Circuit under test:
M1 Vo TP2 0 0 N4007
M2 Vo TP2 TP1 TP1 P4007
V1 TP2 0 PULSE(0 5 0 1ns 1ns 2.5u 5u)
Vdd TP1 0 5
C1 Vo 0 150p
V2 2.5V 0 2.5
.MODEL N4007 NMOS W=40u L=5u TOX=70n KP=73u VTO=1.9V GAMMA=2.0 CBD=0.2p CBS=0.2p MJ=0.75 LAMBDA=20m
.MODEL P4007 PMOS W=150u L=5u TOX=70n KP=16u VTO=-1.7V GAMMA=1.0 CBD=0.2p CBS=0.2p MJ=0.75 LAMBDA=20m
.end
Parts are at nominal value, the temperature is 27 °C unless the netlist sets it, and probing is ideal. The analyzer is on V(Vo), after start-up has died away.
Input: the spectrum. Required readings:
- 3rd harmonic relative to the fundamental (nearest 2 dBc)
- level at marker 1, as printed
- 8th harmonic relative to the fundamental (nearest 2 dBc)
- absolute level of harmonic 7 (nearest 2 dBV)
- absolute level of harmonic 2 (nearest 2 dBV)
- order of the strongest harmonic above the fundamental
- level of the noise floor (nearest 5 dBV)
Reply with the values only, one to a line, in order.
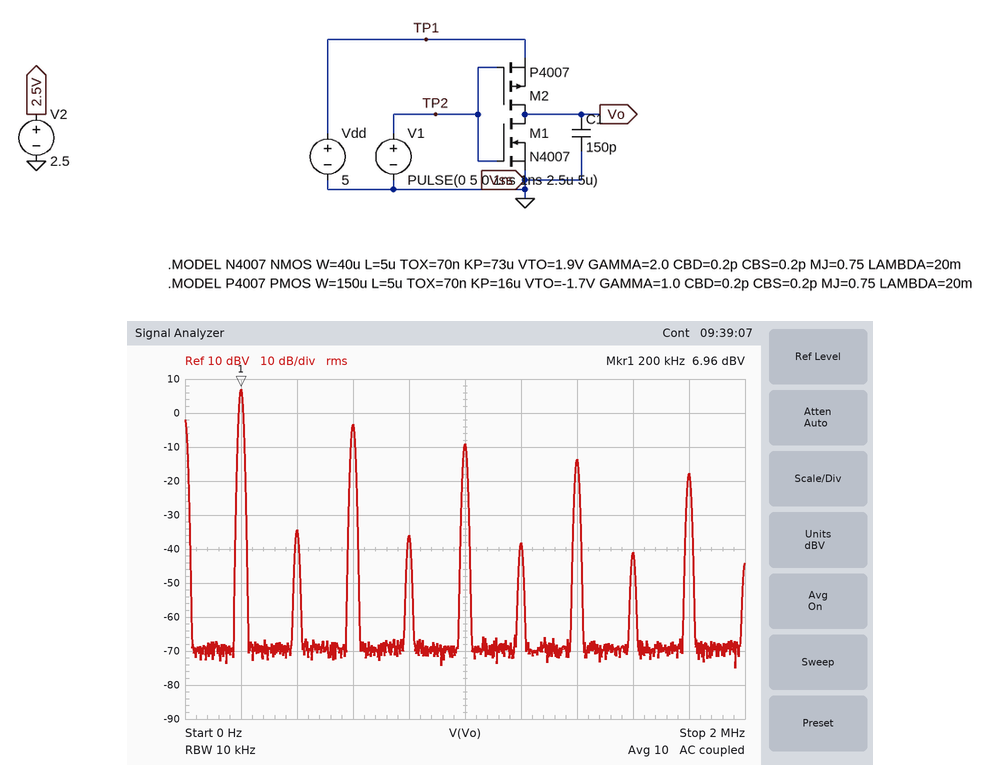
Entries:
-10 dBc
6.96 dBV
-48 dBc
-14 dBV
-34 dBV
3
-70 dBV
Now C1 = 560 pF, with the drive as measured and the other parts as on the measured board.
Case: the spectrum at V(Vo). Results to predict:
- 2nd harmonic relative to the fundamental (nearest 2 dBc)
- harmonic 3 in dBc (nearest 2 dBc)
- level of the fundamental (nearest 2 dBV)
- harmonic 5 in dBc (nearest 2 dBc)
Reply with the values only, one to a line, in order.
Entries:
-34 dBc
-16 dBc
6 dBV
-28 dBc
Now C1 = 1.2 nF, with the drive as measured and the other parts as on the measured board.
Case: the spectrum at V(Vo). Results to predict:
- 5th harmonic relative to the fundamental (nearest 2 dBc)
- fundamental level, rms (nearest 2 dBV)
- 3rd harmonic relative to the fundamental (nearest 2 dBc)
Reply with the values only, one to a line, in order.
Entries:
-30 dBc
2 dBV
-22 dBc
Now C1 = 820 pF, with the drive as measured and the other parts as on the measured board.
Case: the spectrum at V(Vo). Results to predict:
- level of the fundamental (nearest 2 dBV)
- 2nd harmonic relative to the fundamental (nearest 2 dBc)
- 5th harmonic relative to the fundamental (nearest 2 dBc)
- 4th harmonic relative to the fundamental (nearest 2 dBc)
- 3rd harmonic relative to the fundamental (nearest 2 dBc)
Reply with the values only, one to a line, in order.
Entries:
4 dBV
-34 dBc
-30 dBc
-54 dBc
-20 dBc
